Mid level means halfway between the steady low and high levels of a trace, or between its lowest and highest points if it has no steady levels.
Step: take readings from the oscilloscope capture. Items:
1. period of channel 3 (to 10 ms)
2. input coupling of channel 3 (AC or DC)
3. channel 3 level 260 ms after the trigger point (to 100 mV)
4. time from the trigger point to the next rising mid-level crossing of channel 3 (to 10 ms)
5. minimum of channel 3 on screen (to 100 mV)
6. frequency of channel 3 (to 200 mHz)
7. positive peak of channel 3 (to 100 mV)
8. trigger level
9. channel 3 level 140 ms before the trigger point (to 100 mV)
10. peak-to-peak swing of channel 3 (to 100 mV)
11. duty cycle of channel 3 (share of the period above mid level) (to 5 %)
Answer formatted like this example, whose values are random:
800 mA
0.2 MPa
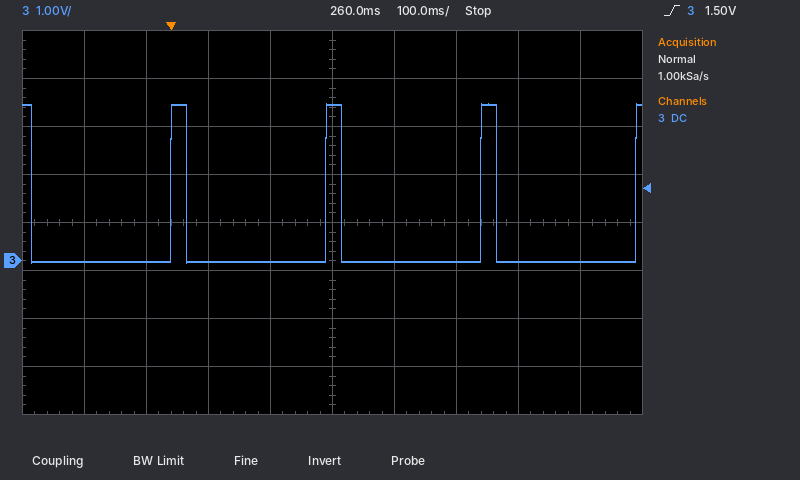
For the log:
250 ms
DC
3.3 V
250 ms
0.0 V
4.0 Hz
3.3 V
1.50 V
0.0 V
3.3 V
10 %
